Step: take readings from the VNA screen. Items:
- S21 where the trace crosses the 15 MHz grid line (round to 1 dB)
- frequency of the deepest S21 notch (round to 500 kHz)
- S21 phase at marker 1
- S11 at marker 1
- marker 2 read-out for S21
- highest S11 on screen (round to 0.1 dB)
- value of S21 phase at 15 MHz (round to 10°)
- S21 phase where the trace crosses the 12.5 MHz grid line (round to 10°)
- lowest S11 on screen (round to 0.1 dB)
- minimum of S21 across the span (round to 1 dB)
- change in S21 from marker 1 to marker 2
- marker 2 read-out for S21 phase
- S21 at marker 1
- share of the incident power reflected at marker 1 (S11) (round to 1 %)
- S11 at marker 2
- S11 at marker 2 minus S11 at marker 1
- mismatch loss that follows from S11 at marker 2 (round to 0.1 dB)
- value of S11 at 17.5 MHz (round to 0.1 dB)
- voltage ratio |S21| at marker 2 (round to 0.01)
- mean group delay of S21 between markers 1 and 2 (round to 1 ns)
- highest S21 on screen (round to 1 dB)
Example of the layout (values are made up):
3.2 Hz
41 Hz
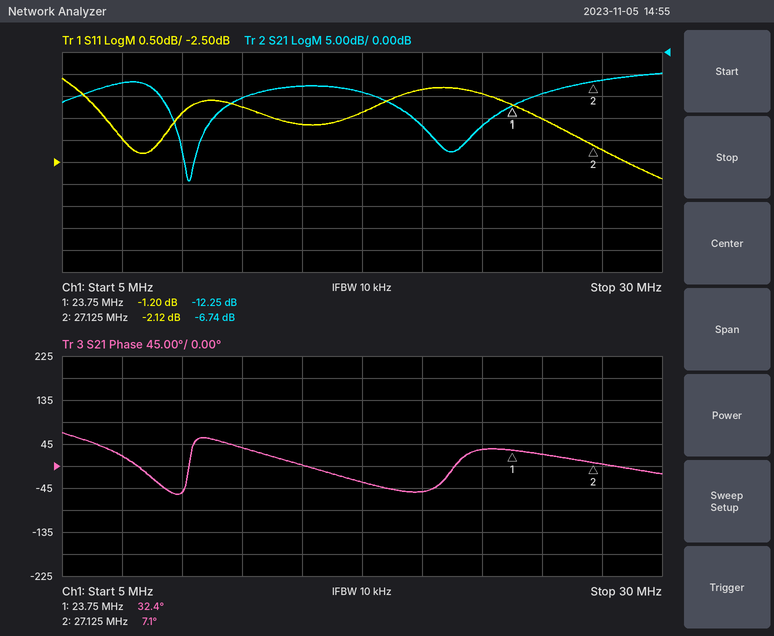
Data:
-8 dB
10.5 MHz
32.4°
-1.20 dB
-6.74 dB
-0.6 dB
0°
40°
-2.9 dB
-29 dB
5.51 dB
7.1°
-12.25 dB
76 %
-2.12 dB
-0.92 dB
4.1 dB
-1.4 dB
0.46
21 ns
-5 dB
